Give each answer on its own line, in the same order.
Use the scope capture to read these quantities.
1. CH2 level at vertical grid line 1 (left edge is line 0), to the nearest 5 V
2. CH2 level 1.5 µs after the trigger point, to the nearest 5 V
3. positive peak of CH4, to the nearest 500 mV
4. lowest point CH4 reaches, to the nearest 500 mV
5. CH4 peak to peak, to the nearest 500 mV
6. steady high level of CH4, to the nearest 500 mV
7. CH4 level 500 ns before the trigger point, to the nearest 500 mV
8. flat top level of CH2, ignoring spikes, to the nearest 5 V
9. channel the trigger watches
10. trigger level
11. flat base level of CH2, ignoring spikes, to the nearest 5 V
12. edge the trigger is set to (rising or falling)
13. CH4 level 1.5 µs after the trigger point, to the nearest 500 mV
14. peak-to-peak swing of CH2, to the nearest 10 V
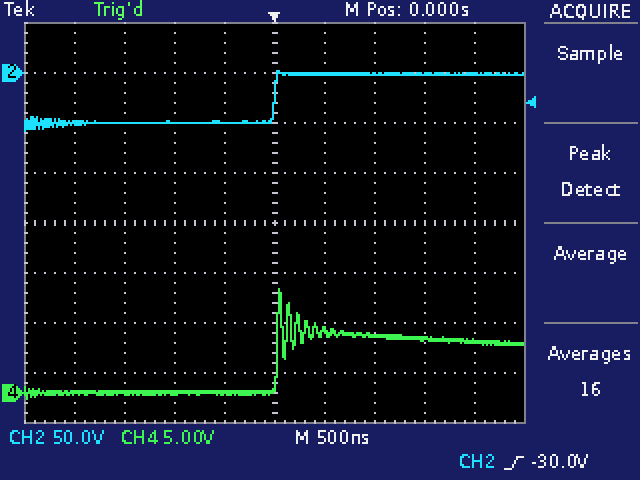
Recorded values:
-50 V
0 V
10.5 V
-500 mV
11.0 V
5.5 V
0.0 V
0 V
CH2
-30.0 V
-50 V
rising
5.5 V
60 V
